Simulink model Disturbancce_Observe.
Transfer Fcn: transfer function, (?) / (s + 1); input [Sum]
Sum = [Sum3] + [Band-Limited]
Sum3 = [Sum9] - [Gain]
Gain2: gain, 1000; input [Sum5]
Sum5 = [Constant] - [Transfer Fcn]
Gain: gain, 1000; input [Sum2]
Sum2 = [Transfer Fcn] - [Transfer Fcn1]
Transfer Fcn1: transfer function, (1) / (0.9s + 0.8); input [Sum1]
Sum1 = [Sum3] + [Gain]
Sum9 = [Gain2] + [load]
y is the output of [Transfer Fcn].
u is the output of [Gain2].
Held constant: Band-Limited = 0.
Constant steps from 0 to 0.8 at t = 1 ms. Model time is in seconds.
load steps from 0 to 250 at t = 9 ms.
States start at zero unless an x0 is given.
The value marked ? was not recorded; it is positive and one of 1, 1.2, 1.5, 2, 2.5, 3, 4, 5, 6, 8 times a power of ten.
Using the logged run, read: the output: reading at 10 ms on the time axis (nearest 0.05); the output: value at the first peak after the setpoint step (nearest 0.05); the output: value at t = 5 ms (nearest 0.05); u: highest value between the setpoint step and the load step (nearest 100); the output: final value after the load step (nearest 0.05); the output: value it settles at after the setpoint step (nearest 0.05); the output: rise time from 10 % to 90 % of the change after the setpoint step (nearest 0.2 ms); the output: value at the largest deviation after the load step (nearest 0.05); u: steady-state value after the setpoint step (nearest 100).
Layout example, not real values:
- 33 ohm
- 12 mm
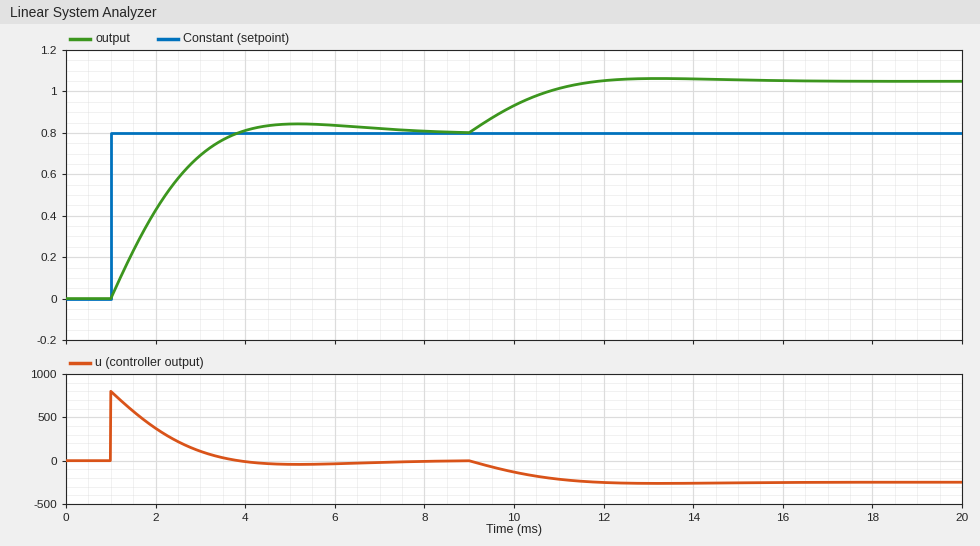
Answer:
- 0.95
- 0.85
- 0.85
- 800
- 1.05
- 0.80
- 2.0 ms
- 1.05
- 0
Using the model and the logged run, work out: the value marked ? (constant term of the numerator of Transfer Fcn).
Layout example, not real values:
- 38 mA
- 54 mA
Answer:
- 0.6
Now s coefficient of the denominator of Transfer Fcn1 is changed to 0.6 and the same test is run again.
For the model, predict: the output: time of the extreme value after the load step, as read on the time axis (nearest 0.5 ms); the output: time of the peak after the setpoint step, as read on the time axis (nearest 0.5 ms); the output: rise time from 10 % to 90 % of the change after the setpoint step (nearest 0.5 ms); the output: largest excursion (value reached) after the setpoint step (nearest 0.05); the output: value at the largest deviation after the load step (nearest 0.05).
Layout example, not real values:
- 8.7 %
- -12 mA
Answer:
- 12.0 ms
- 4.0 ms
- 1.5 ms
- 0.90
- 1.10
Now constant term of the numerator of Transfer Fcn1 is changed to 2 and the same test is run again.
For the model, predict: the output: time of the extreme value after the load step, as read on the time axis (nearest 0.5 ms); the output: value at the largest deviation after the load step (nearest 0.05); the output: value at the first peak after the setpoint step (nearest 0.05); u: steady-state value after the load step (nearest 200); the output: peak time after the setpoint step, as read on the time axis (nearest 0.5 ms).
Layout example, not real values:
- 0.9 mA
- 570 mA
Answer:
- 11.5 ms
- 1.10
- 0.95
- -200
- 3.5 ms
